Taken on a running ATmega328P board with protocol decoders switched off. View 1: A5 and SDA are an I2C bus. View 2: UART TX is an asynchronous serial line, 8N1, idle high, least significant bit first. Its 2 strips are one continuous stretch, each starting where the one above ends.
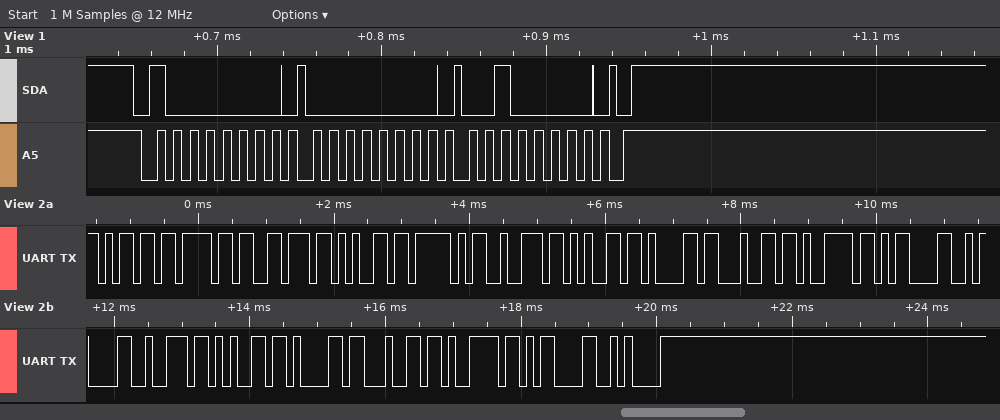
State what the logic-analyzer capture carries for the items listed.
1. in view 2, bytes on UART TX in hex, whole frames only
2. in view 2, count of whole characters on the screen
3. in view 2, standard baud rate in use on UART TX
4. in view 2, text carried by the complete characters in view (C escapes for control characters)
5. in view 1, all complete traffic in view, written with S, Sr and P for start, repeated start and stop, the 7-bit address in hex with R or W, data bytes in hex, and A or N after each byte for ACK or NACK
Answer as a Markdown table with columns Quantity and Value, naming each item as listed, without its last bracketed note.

| Quantity | Value |
|---|---|
| in view 2, bytes on UART TX in hex, whole frames only | 0x6D 0x6F 0x76 0x65 0x5F 0x72 0x65 0x61 0x64 0x79 0x0D 0x0A 0x72 0x65 0x61 0x64 0x79 0x0D 0x0A |
| in view 2, count of whole characters on the screen | 19 |
| in view 2, standard baud rate in use on UART TX | 9600 baud |
| in view 2, text carried by the complete characters in view | "move_ready\r\nready\r\n" |
| in view 1, all complete traffic in view, written with S, Sr and P for start, repeated start and stop, the 7-bit address in hex with R or W, data bytes in hex, and A or N after each byte for ACK or NACK | S 40W A 00 A 20 A P |
